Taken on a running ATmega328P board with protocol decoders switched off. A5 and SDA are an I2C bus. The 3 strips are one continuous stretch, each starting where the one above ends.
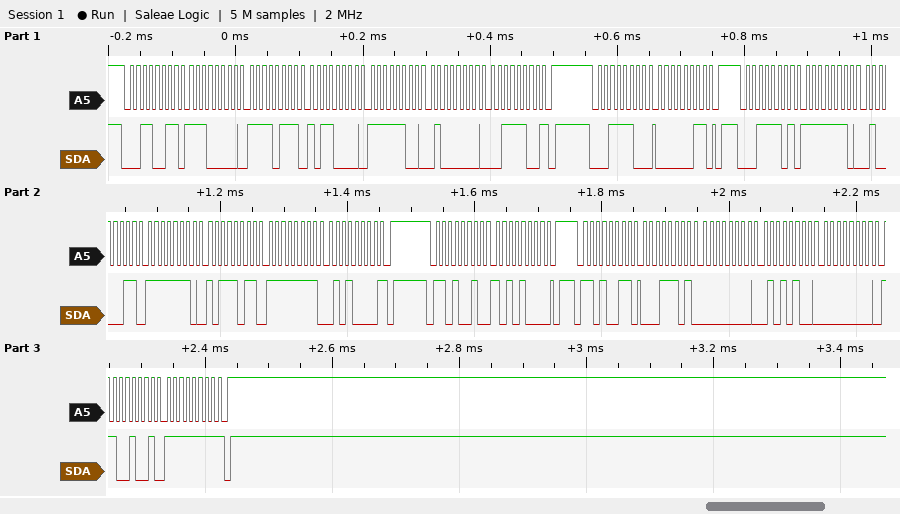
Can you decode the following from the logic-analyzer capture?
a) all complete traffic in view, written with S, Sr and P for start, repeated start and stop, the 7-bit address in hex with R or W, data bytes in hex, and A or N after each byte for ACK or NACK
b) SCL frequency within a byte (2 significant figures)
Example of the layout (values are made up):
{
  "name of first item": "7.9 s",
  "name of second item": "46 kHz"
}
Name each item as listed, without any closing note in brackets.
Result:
{
  "all complete traffic in view, written with S, Sr and P for start, repeated start and stop, the 7-bit address in hex with R or W, data bytes in hex, and A or N after each byte for ACK or NACK": "S 19R A E0 A F7 A B0 A FC A 40 A 3C N P S 1EW A 03 A P S 1ER A FE A 43 A FE A BB A FF A 50 N P S 69W A A8 A P S 69R A 1D A 00 A 54 A 00 A C9 A FF N P",
  "SCL frequency within a byte": "100 kHz"
}
